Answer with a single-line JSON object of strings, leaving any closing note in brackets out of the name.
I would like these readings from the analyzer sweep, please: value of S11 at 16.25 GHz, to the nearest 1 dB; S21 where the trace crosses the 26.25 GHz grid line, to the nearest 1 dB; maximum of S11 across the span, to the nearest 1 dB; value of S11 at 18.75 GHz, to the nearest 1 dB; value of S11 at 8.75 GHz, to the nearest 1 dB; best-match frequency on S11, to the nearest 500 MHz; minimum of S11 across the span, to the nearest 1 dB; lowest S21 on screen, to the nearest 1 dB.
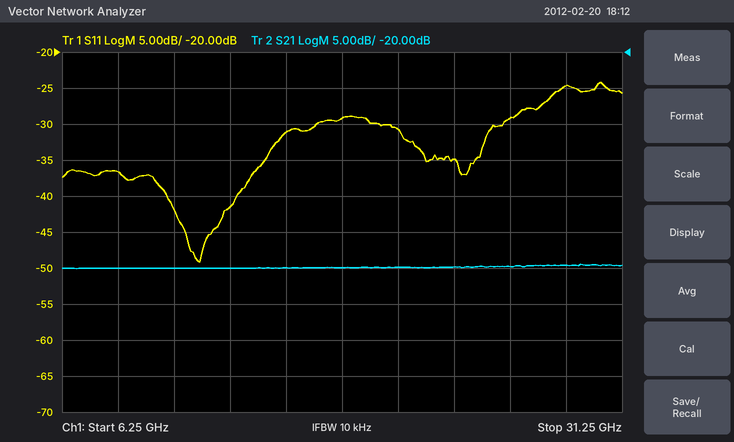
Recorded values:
{"value of S11 at 16.25 GHz, to the nearest 1 dB": "-31 dB", "S21 where the trace crosses the 26.25 GHz grid line, to the nearest 1 dB": "-50 dB", "maximum of S11 across the span, to the nearest 1 dB": "-24 dB", "value of S11 at 18.75 GHz, to the nearest 1 dB": "-29 dB", "value of S11 at 8.75 GHz, to the nearest 1 dB": "-37 dB", "best-match frequency on S11, to the nearest 500 MHz": "12.5 GHz", "minimum of S11 across the span, to the nearest 1 dB": "-49 dB", "lowest S21 on screen, to the nearest 1 dB": "-50 dB"}
